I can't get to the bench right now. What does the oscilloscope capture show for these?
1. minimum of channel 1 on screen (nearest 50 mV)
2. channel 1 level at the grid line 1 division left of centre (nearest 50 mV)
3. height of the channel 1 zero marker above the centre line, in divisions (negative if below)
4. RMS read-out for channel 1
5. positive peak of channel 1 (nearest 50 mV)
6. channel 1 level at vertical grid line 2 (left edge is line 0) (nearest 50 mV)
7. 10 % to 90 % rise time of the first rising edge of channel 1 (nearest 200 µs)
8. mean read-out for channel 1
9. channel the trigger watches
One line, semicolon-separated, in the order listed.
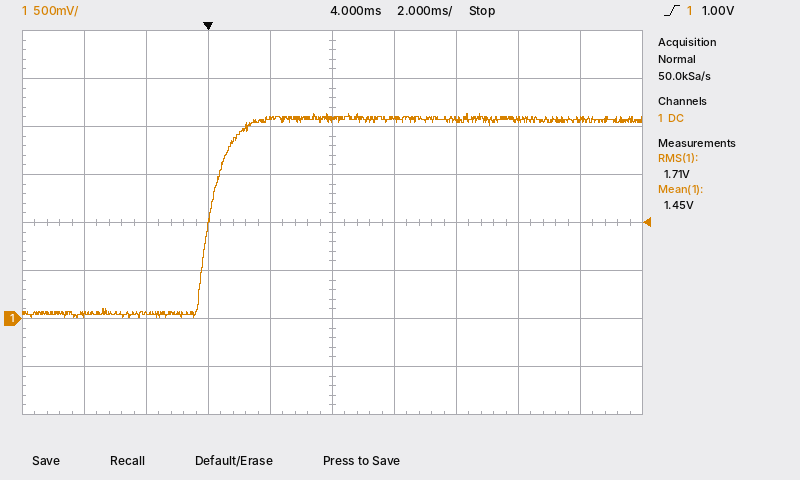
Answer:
0 mV; 2.10 V; -2.0 div; 1.71 V; 2.15 V; 50 mV; 1.2 ms; 1.45 V; channel 1
